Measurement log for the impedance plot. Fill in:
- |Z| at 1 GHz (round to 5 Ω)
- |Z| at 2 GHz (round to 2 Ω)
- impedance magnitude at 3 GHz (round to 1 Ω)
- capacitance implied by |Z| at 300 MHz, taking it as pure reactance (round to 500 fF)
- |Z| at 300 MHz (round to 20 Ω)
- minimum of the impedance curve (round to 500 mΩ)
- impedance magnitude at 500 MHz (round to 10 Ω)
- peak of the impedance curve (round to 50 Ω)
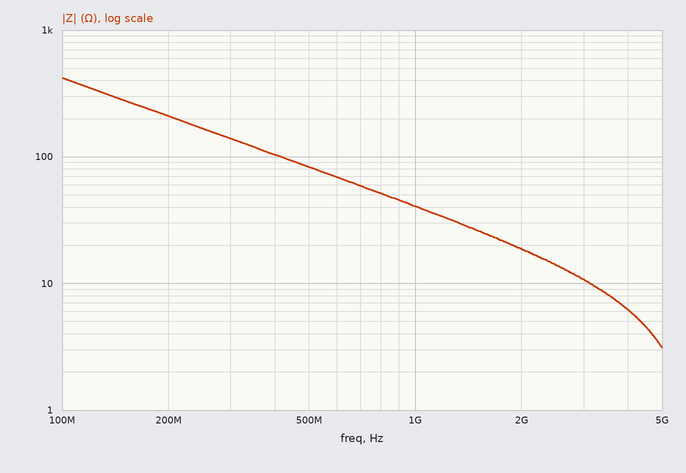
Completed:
40 Ω
18 Ω
11 Ω
4.0 pF
140 Ω
3.0 Ω
80 Ω
400 Ω
